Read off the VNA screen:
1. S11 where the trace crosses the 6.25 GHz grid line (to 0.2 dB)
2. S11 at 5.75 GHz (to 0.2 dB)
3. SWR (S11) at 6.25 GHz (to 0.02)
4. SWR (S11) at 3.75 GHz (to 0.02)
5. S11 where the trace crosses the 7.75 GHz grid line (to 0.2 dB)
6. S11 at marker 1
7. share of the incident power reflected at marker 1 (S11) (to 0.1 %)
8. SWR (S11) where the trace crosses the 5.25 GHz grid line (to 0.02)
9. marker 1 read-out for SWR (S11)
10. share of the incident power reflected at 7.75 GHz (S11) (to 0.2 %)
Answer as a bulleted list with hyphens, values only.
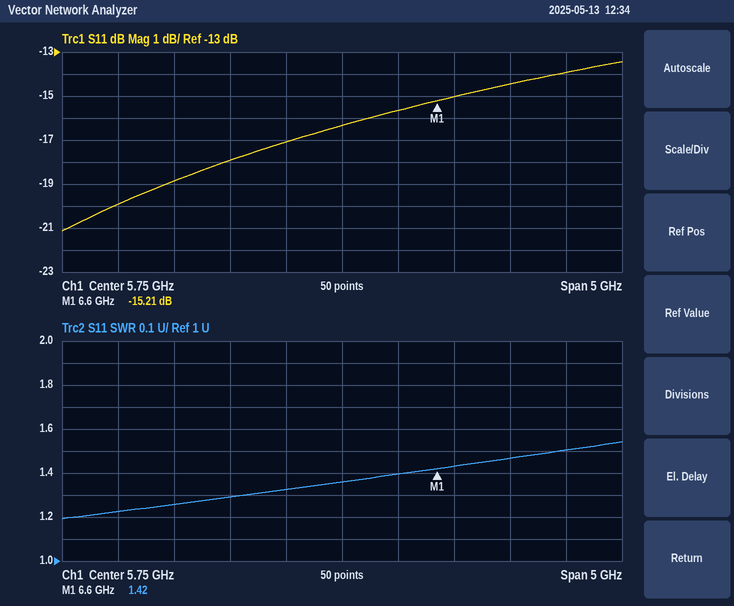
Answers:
- -15.6 dB
- -16.4 dB
- 1.40
- 1.22
- -14.0 dB
- -15.21 dB
- 3.0 %
- 1.32
- 1.42
- 4.0 %
